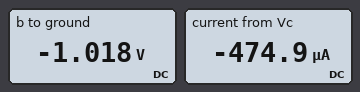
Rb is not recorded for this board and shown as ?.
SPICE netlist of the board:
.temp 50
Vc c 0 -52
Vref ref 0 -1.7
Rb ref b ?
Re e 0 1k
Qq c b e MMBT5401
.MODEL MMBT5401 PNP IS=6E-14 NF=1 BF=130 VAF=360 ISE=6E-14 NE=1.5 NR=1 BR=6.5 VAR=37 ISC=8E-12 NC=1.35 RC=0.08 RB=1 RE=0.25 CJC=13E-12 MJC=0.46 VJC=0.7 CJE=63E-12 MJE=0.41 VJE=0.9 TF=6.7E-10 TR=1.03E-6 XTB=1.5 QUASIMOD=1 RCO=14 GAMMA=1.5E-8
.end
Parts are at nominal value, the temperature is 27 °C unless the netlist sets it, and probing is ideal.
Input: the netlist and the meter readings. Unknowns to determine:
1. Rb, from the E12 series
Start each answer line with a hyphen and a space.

- 220 kΩ
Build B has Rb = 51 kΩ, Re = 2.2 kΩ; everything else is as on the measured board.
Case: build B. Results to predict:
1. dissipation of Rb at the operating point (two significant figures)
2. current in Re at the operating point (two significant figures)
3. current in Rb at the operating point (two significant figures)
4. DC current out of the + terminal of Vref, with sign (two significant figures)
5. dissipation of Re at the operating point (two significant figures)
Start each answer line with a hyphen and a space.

- 450 nW
- 460 µA
- 3.0 µA
- -3.0 µA
- 460 µW
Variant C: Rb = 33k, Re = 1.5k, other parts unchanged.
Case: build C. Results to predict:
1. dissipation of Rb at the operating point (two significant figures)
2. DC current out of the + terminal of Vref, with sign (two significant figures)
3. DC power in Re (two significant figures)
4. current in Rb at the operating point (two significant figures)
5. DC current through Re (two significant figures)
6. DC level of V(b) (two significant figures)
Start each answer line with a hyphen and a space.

- 620 nW
- -4.3 µA
- 680 µW
- 4.3 µA
- 670 µA
- -1.6 V
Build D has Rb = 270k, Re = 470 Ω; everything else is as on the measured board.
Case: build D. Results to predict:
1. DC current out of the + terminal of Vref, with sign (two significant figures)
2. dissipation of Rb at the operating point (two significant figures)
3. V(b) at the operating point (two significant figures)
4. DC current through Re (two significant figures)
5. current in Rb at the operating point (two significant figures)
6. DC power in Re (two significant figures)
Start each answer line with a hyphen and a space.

- -3.4 µA
- 3.1 µW
- -790 mV
- 520 µA
- 3.4 µA
- 130 µW
